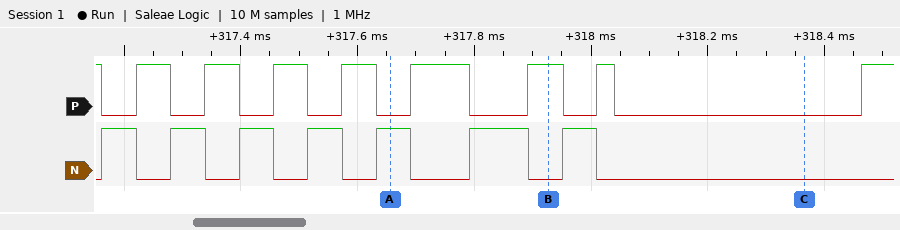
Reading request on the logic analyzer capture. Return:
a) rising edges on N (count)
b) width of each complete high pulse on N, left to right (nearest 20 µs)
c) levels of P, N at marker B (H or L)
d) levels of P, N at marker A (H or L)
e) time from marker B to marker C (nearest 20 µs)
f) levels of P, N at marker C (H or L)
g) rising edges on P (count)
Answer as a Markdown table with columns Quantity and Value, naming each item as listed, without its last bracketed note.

| Quantity | Value |
|---|---|
| rising edges on N | 7 |
| width of each complete high pulse on N, left to right | 60 µs, 60 µs, 60 µs, 60 µs, 60 µs, 100 µs, 60 µs |
| levels of P, N at marker B | P=H, N=L |
| levels of P, N at marker A | P=L, N=H |
| time from marker B to marker C | 440 µs |
| levels of P, N at marker C | P=L, N=L |
| rising edges on P | 8 |
